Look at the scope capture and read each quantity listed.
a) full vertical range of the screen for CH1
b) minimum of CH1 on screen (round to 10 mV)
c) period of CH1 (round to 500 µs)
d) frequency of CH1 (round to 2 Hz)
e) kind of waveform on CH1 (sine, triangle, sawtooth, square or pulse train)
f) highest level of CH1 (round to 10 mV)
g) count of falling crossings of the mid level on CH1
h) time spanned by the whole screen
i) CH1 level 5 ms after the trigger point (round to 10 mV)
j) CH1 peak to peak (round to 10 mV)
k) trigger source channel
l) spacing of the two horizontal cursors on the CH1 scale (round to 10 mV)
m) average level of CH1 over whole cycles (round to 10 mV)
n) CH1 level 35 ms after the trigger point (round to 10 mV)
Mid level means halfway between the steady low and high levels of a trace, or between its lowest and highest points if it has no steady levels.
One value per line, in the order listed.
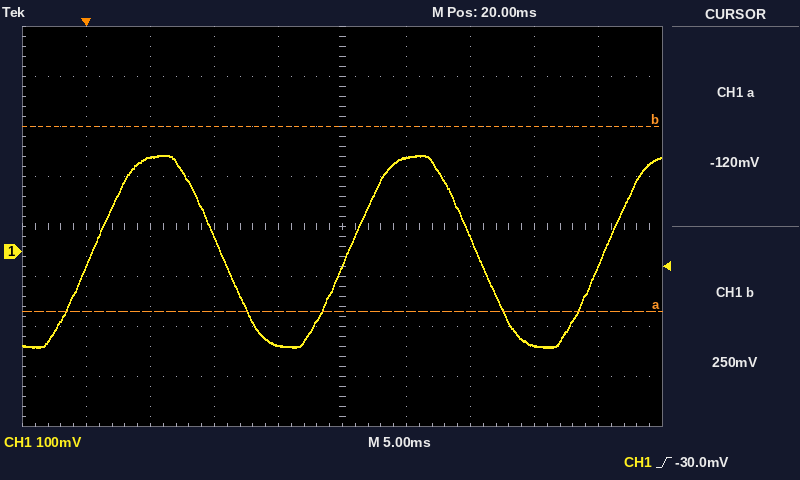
800 mV
-190 mV
20.0 ms
50 Hz
sine
190 mV
2
50 ms
190 mV
380 mV
CH1
370 mV
0 mV
-190 mV
